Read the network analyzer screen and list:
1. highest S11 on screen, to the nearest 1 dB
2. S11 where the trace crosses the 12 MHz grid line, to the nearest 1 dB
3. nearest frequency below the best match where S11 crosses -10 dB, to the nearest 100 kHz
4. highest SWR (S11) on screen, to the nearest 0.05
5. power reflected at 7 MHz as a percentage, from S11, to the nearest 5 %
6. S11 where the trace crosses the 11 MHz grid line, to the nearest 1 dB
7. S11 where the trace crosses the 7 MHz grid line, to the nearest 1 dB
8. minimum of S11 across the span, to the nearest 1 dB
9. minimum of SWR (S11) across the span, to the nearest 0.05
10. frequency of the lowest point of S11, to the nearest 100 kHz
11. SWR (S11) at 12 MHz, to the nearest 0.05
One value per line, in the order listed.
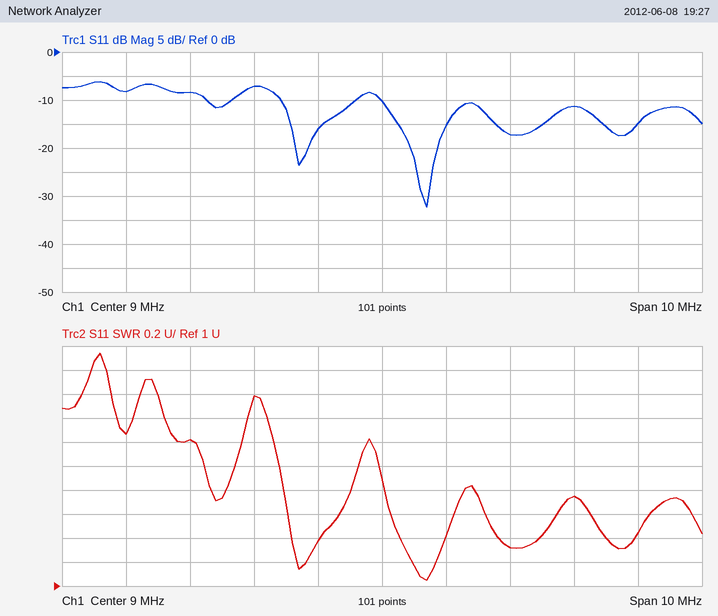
-6 dB
-11 dB
9.0 MHz
2.95
20 %
-17 dB
-7 dB
-32 dB
1.05
9.7 MHz
1.75
